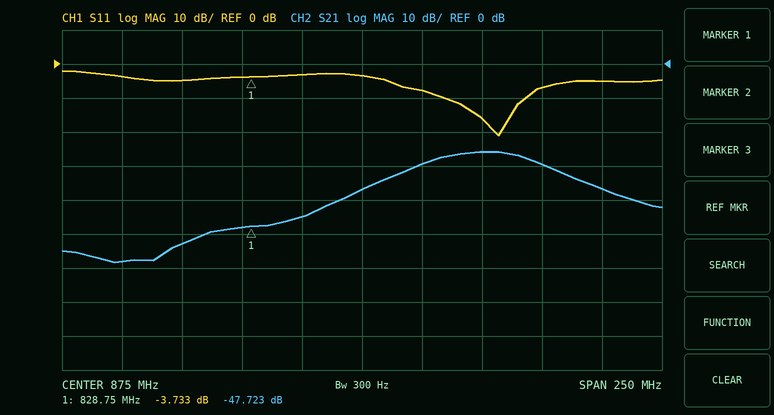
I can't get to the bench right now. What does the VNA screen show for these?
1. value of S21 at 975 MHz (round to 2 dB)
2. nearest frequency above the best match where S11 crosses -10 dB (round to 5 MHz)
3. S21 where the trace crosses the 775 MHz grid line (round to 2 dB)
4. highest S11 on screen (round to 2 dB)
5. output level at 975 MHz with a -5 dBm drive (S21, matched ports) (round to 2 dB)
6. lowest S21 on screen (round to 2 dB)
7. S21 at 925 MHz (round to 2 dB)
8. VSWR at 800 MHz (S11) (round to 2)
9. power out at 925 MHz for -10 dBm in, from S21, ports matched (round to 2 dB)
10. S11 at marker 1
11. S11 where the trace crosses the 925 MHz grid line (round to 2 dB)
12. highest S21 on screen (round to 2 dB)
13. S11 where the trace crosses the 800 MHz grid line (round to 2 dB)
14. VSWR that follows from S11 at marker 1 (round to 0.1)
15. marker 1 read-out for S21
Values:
-36 dB
945 MHz
-58 dB
-2 dB
-42 dBm
-58 dB
-26 dB
4
-36 dBm
-3.733 dB
-16 dB
-26 dB
-4 dB
4.7
-47.723 dB
